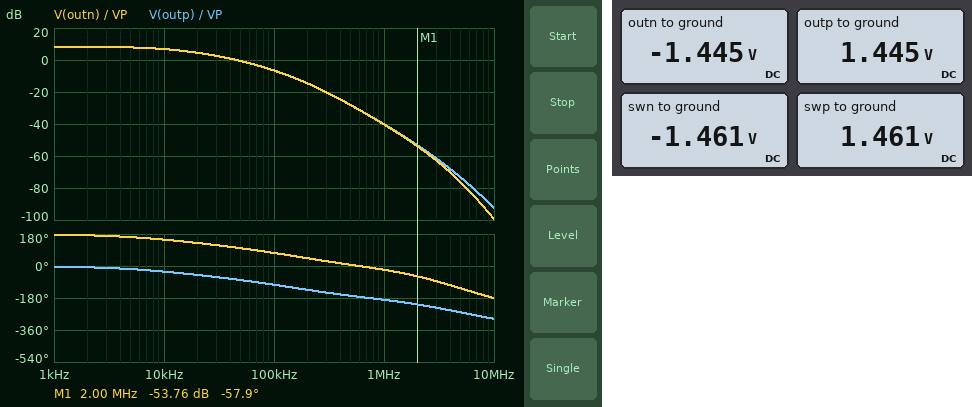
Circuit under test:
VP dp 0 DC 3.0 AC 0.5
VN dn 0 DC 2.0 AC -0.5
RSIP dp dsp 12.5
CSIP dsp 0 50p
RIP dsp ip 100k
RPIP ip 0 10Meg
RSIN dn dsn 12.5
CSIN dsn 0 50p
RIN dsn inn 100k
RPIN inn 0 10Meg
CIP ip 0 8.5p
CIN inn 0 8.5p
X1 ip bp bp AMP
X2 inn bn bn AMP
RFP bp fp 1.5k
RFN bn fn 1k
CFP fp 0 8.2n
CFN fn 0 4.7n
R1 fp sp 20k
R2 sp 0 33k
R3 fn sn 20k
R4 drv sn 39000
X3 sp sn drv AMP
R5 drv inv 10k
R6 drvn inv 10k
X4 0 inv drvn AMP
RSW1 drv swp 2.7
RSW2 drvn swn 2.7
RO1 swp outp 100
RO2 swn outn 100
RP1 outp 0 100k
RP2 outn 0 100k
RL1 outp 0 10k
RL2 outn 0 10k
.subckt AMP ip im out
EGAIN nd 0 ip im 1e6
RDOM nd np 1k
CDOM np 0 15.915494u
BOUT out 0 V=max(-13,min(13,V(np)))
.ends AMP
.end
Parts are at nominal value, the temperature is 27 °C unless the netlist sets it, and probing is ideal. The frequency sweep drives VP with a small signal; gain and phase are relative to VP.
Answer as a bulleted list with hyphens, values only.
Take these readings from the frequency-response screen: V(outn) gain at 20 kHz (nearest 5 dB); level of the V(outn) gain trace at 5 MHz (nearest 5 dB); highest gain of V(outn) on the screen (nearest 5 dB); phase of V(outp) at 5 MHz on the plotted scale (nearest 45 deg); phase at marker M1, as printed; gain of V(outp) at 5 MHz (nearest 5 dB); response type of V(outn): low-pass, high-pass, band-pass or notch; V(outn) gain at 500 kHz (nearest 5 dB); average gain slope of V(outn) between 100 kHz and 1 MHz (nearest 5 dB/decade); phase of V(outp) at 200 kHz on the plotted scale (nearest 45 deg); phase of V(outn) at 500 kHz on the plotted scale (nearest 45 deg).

- 5 dB
- -75 dB
- 10 dB
- -270 deg
- -57.9 deg
- -75 dB
- low-pass
- -30 dB
- -35 dB/decade
- -135 deg
- 0 deg
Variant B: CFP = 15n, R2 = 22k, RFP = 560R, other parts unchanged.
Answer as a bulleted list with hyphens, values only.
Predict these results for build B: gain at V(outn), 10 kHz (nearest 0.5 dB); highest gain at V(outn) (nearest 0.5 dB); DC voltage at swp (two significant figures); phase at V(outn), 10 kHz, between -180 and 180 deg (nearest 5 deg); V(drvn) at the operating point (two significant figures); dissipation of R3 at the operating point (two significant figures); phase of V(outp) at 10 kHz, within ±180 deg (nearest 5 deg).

- 6.5 dB
- 7.5 dB
- 710 mV
- 155 deg
- -710 mV
- 9.0 µW
- -25 deg
